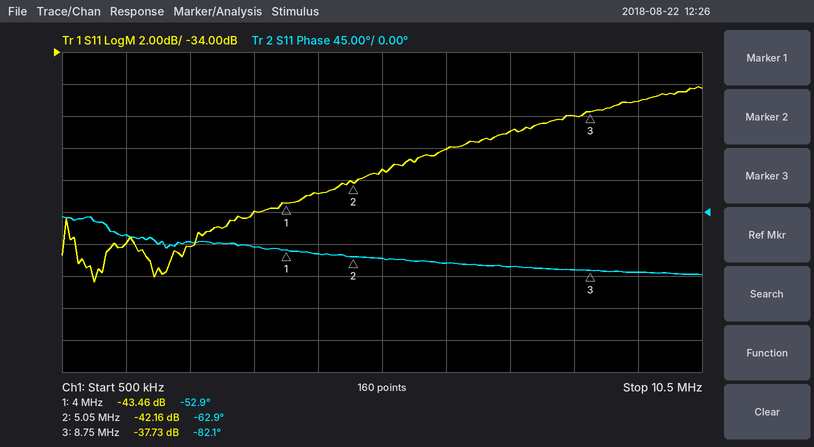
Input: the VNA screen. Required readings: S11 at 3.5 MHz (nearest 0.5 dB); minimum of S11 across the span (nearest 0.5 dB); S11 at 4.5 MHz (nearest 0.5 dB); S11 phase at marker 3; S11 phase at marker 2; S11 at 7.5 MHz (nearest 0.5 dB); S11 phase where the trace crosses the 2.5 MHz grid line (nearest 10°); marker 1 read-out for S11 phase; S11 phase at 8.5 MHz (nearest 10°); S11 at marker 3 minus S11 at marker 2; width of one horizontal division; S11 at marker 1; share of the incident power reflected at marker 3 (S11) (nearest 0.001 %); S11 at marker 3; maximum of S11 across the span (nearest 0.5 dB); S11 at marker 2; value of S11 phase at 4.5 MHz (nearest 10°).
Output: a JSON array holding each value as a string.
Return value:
["-44.0 dB", "-48.5 dB", "-43.0 dB", "-82.1°", "-62.9°", "-39.0 dB", "-40°", "-52.9°", "-80°", "4.43 dB", "1 MHz", "-43.46 dB", "0.017 %", "-37.73 dB", "-36.0 dB", "-42.16 dB", "-60°"]
